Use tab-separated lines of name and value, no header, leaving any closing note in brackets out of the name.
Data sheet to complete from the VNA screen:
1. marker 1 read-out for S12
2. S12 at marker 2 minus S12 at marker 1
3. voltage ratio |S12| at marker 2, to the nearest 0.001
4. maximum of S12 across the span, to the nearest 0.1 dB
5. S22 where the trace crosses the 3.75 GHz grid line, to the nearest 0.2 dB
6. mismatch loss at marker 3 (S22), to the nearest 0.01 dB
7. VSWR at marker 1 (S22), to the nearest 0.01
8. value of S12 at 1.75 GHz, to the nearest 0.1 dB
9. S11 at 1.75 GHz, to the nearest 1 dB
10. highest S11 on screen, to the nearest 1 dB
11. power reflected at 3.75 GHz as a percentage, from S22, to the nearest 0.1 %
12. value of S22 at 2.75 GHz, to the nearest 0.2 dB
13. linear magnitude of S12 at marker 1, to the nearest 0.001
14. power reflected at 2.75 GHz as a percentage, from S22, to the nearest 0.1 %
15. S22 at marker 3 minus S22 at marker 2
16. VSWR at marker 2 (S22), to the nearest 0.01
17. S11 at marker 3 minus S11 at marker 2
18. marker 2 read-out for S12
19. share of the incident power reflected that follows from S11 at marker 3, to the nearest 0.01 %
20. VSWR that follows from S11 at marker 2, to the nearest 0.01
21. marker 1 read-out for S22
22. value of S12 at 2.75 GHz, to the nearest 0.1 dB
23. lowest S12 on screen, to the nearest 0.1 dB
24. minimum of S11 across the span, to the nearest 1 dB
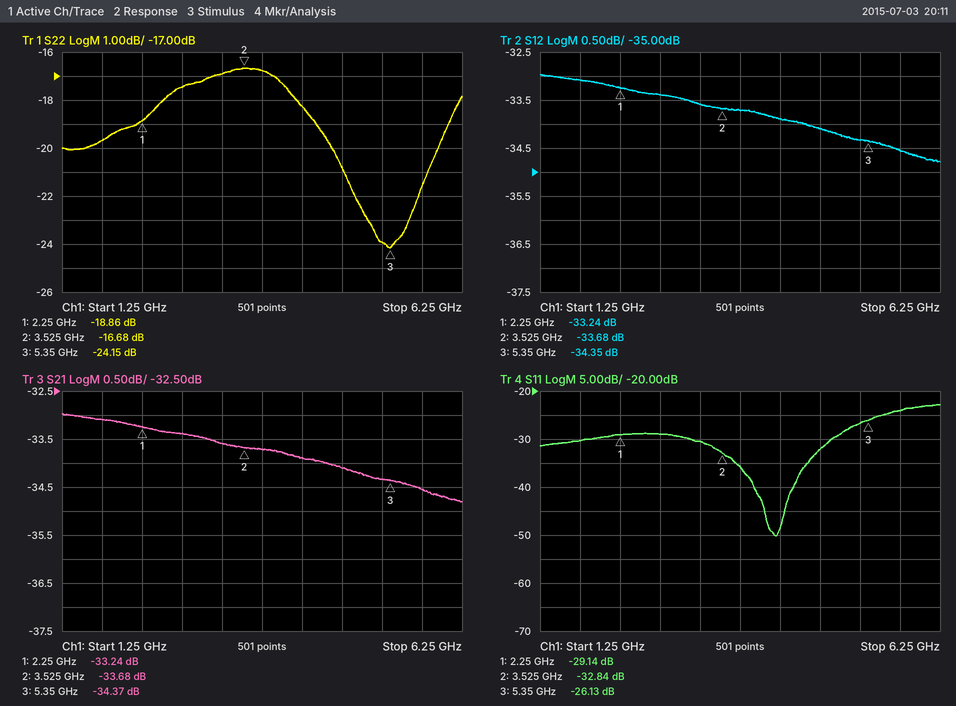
marker 1 read-out for S12	-33.24 dB
S12 at marker 2 minus S12 at marker 1	-0.44 dB
voltage ratio |S12| at marker 2, to the nearest 0.001	0.021
maximum of S12 across the span, to the nearest 0.1 dB	-33.0 dB
S22 where the trace crosses the 3.75 GHz grid line, to the nearest 0.2 dB	-16.8 dB
mismatch loss at marker 3 (S22), to the nearest 0.01 dB	0.02 dB
VSWR at marker 1 (S22), to the nearest 0.01	1.26
value of S12 at 1.75 GHz, to the nearest 0.1 dB	-33.1 dB
S11 at 1.75 GHz, to the nearest 1 dB	-30 dB
highest S11 on screen, to the nearest 1 dB	-23 dB
power reflected at 3.75 GHz as a percentage, from S22, to the nearest 0.1 %	2.1 %
value of S22 at 2.75 GHz, to the nearest 0.2 dB	-17.4 dB
linear magnitude of S12 at marker 1, to the nearest 0.001	0.022
power reflected at 2.75 GHz as a percentage, from S22, to the nearest 0.1 %	1.8 %
S22 at marker 3 minus S22 at marker 2	-7.47 dB
VSWR at marker 2 (S22), to the nearest 0.01	1.34
S11 at marker 3 minus S11 at marker 2	6.71 dB
marker 2 read-out for S12	-33.68 dB
share of the incident power reflected that follows from S11 at marker 3, to the nearest 0.01 %	0.24 %
VSWR that follows from S11 at marker 2, to the nearest 0.01	1.05
marker 1 read-out for S22	-18.86 dB
value of S12 at 2.75 GHz, to the nearest 0.1 dB	-33.4 dB
lowest S12 on screen, to the nearest 0.1 dB	-34.8 dB
minimum of S11 across the span, to the nearest 1 dB	-50 dB
